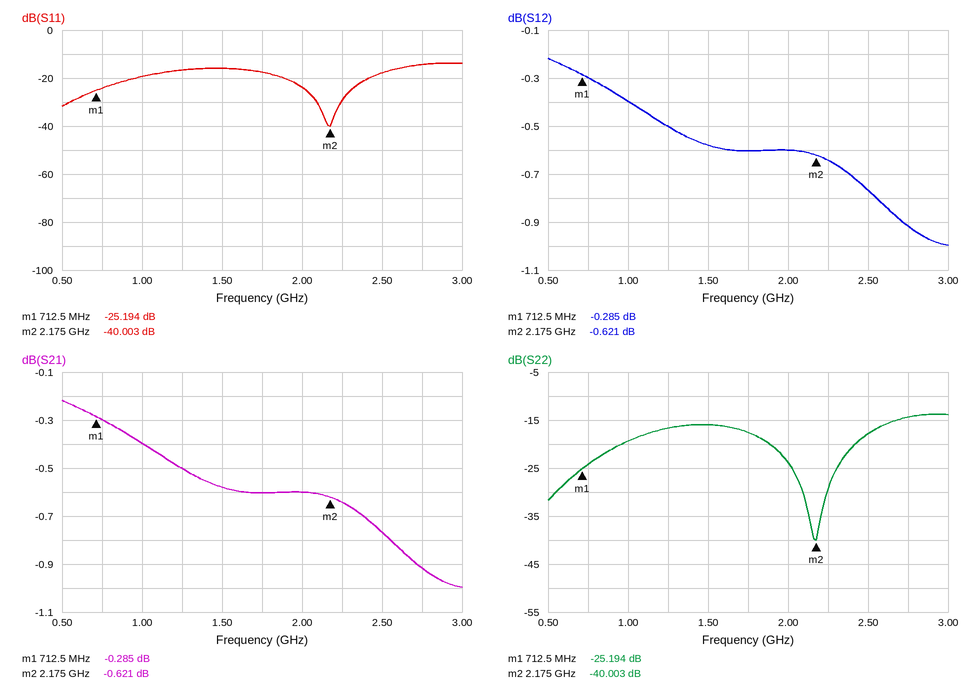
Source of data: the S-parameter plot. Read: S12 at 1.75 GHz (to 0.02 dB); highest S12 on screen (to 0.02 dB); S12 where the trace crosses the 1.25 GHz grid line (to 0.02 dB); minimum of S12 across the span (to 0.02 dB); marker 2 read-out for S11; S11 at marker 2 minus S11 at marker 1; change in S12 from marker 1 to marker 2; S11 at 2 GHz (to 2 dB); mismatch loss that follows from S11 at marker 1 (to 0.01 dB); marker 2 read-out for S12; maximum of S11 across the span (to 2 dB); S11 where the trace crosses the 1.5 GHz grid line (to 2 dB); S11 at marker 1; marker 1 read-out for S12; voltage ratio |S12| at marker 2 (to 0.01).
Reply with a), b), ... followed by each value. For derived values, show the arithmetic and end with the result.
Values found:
a) -0.60 dB
b) -0.22 dB
c) -0.50 dB
d) -1.00 dB
e) -40.003 dB
f) -40.003 − (-25.194) = -14.809 dB
g) -0.621 − (-0.285) = -0.336 dB
h) -24 dB
i) −10 log10(1 − 10^(-25.194/10)) ≈ 0.01 dB
j) -0.621 dB
k) -14 dB
l) -16 dB
m) -25.194 dB
n) -0.285 dB
o) 10^(-0.621/20) ≈ 0.93
